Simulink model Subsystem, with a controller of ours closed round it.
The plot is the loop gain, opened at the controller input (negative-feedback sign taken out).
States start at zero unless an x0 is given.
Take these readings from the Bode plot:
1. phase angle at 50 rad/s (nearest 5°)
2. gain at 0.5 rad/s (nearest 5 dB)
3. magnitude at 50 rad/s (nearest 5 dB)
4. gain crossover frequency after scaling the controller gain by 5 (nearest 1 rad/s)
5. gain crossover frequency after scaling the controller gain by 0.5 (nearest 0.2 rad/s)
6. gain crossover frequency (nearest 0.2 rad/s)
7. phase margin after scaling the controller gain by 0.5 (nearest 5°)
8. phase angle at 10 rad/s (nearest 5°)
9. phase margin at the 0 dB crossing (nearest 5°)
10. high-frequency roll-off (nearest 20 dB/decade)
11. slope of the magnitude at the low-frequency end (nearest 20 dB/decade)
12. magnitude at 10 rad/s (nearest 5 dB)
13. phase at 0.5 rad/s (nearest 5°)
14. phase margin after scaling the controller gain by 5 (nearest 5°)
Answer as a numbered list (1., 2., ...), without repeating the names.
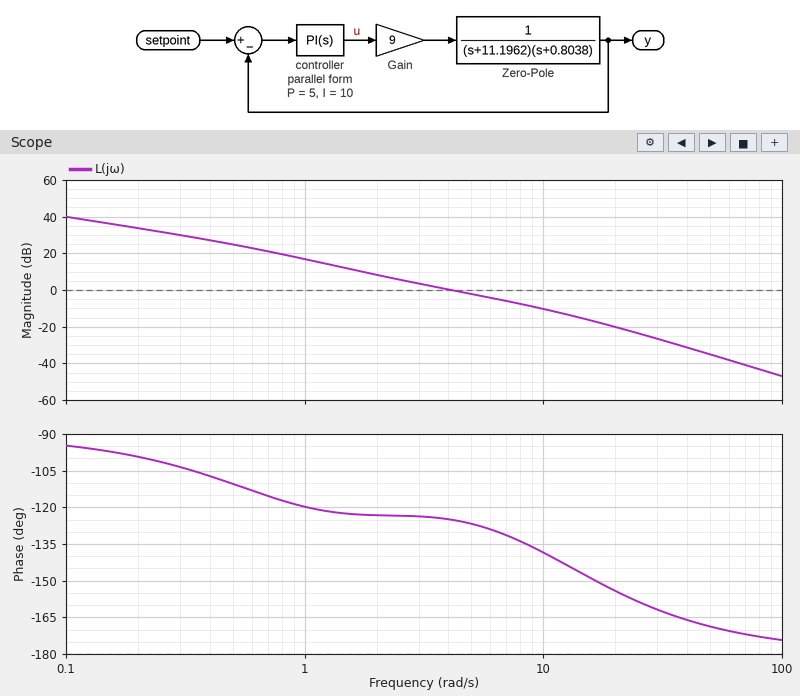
1. -170°
2. 25 dB
3. -35 dB
4. 13 rad/s
5. 2.4 rad/s
6. 4.2 rad/s
7. 55°
8. -140°
9. 55°
10. -40 dB/decade
11. -20 dB/decade
12. -10 dB
13. -110°
14. 35°
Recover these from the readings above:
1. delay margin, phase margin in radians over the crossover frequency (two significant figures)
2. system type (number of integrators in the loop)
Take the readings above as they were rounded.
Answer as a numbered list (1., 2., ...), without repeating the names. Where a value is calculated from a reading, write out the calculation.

1. 55 × π / 180 / 4.2 = 0.23 s
2. 1
